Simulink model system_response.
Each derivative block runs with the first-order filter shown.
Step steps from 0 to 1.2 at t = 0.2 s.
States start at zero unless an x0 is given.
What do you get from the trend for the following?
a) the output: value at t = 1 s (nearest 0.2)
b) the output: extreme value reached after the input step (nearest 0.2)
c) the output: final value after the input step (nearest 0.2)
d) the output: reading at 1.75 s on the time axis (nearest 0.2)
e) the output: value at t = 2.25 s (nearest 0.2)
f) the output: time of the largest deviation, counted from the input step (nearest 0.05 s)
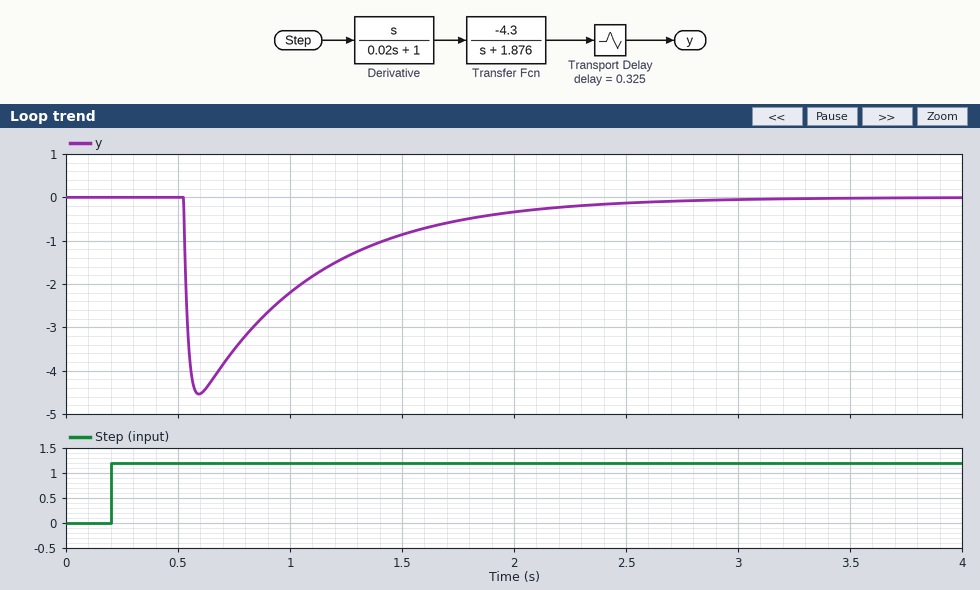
-2.2
-4.6
0.0
-0.6
-0.2
0.40 s
